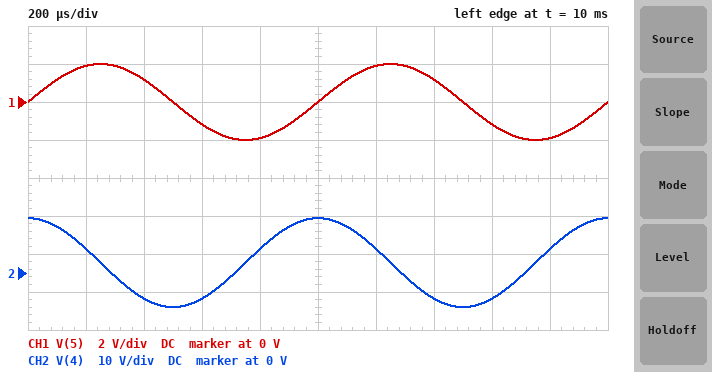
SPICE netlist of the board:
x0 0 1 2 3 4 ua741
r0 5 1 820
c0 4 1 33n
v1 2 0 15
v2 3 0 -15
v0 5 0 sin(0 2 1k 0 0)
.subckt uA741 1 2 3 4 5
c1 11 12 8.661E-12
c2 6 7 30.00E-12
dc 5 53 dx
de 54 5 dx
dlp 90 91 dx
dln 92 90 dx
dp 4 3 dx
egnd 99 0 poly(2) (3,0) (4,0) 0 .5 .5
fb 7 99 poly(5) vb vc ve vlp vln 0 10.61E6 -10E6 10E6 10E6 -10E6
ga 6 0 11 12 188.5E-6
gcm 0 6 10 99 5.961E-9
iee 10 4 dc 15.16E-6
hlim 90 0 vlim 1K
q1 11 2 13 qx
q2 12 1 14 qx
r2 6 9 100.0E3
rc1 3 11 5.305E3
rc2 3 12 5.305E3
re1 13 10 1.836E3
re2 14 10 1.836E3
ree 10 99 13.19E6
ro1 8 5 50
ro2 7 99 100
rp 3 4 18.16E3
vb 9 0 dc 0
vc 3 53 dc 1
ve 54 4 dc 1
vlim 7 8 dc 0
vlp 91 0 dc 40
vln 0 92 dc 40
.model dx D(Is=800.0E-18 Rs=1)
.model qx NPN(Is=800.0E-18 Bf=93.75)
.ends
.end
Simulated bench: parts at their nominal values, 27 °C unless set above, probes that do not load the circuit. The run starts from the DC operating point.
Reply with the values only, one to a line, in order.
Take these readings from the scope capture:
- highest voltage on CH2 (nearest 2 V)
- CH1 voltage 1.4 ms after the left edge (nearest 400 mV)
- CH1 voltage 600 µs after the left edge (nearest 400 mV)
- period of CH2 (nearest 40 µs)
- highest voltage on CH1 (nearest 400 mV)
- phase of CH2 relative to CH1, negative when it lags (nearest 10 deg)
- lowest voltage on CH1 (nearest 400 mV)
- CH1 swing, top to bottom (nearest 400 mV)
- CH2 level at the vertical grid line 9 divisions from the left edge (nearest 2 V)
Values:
14 V
1.2 V
-1.2 V
1.00 ms
2.0 V
90 deg
-2.0 V
4.0 V
6 V
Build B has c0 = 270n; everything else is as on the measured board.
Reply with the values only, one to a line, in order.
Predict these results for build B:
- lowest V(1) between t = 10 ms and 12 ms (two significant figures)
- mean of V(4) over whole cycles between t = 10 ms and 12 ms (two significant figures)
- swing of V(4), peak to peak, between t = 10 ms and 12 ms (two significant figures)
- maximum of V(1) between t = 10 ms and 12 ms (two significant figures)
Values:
-1.5 mV
13 V
2.9 V
1.4 mV
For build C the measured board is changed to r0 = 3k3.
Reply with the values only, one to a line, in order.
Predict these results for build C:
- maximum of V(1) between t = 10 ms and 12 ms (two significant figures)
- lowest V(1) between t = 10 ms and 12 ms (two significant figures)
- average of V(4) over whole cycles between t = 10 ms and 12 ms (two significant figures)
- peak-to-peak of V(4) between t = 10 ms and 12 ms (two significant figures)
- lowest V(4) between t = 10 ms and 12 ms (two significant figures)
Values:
2.9 mV
-3.0 mV
12 V
5.8 V
8.6 V
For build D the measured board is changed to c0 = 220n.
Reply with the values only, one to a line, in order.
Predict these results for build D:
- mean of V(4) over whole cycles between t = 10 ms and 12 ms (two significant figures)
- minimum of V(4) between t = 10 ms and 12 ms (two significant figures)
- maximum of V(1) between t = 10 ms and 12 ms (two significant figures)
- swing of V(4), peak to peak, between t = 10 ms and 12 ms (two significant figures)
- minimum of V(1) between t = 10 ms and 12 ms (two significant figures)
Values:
13 V
11 V
1.7 mV
3.5 V
-1.8 mV
